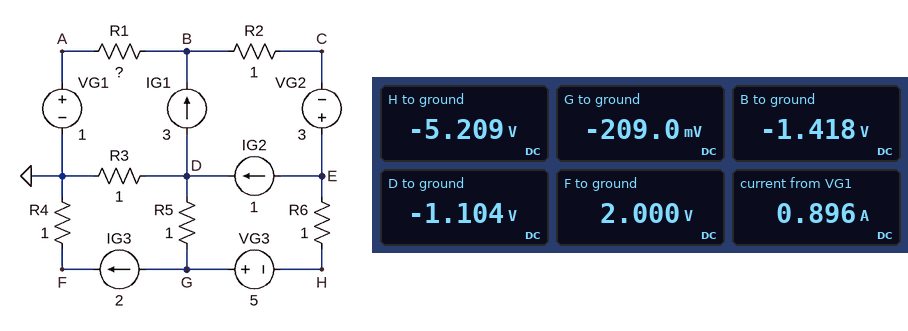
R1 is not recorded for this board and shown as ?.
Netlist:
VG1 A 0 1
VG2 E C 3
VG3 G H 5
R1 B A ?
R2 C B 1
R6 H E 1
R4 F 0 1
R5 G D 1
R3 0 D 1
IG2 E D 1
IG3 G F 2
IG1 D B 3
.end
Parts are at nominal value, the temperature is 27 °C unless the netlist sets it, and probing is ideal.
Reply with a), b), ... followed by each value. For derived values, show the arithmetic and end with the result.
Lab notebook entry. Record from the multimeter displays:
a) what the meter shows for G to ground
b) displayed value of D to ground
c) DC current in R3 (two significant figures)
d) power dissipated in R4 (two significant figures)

a) -209.0 mV
b) -1.104 V
c) (0 V - (-1.104 V)) / 1 Ω = 1.1 A
d) (2 V)^2 / 1 Ω = 4.0 W
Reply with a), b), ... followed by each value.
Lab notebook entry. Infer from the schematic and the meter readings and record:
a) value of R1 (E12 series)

a) 2.7 Ω
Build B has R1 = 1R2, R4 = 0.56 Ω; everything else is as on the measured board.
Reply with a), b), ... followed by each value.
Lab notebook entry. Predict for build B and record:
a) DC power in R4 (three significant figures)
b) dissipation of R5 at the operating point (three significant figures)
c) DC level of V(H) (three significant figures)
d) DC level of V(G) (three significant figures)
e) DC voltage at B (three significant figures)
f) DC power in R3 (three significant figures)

a) 2.24 W
b) 1.33 W
c) -4.69 V
d) 308 mV
e) -385 mV
f) 716 mW
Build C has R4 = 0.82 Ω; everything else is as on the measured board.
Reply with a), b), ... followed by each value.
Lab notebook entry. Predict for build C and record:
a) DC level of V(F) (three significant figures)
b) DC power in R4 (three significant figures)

a) 1.64 V
b) 3.28 W
